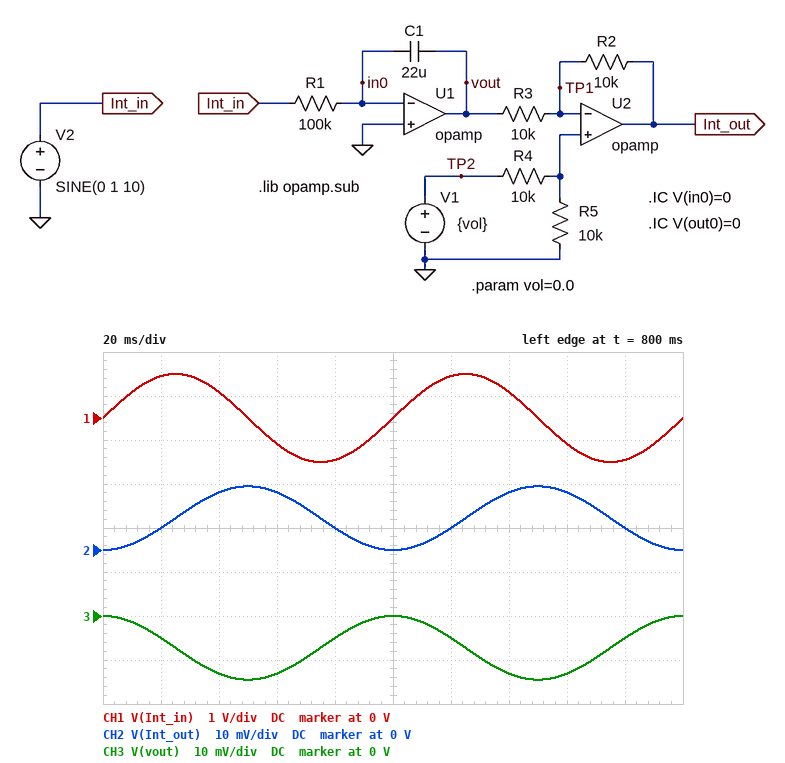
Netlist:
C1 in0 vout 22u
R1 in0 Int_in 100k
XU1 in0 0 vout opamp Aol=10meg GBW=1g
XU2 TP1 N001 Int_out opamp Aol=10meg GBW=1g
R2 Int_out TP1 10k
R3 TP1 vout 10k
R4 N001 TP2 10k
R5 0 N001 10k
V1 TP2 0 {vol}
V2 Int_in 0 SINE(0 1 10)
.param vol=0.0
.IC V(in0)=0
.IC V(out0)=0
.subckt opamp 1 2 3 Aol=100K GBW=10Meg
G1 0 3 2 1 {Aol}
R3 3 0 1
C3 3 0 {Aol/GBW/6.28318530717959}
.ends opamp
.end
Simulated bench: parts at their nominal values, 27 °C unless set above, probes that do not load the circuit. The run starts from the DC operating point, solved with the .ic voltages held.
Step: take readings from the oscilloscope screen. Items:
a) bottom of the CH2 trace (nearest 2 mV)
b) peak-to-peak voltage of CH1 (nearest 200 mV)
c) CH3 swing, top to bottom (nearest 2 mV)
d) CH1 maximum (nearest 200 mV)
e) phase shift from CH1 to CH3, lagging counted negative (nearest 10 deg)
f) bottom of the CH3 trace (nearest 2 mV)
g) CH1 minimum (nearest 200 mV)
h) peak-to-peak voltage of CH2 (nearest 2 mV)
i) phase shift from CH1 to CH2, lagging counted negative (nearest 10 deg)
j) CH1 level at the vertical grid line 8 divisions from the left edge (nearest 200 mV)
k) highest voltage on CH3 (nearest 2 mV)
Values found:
0 V
2.0 V
14 mV
1.0 V
90 deg
-14 mV
-1.0 V
14 mV
-90 deg
-600 mV
0 V
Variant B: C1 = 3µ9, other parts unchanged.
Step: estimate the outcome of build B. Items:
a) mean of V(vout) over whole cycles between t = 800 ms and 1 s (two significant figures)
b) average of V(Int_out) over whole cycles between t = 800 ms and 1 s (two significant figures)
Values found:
-41 mV
41 mV
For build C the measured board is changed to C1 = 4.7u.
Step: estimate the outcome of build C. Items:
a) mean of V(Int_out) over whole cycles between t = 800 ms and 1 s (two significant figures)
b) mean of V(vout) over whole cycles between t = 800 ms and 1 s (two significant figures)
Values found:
34 mV
-34 mV
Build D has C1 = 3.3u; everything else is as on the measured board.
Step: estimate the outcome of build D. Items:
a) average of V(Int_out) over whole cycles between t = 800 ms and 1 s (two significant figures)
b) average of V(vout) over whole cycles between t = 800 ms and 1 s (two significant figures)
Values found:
48 mV
-48 mV
